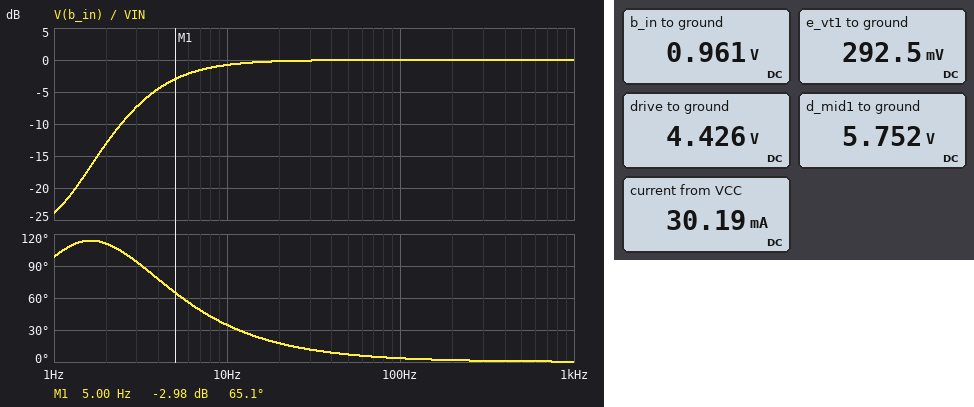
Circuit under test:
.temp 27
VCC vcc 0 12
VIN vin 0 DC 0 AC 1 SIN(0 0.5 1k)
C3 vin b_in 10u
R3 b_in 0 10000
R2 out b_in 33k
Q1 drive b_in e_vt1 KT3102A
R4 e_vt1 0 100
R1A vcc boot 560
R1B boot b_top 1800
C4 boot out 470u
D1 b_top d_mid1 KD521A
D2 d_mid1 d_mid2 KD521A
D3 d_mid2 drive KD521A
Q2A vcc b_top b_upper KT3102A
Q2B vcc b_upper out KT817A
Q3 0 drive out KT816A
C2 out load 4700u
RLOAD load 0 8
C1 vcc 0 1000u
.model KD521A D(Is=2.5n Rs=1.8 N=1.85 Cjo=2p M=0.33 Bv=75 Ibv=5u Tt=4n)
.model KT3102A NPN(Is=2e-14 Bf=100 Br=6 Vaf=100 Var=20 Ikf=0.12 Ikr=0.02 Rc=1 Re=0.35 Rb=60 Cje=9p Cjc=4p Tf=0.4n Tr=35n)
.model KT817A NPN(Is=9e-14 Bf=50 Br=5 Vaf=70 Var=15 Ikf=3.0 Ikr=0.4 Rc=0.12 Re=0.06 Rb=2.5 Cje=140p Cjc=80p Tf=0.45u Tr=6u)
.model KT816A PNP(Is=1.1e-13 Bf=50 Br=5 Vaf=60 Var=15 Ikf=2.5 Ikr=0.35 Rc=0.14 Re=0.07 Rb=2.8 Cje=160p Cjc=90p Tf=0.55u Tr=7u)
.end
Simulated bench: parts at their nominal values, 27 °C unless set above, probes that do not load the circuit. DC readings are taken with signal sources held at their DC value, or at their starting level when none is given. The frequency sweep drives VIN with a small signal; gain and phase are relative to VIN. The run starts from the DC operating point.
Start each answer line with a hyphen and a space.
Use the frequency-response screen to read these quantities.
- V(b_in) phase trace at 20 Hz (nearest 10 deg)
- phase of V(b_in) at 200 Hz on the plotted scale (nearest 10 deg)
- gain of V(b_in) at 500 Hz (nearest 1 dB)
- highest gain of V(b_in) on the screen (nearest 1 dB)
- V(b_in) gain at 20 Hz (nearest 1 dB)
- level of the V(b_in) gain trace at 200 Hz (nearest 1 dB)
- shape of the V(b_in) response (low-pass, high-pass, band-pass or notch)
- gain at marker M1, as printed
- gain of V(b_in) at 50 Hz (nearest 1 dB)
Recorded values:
- 20 deg
- 0 deg
- 0 dB
- 0 dB
- 0 dB
- 0 dB
- high-pass
- -2.98 dB
- 0 dB
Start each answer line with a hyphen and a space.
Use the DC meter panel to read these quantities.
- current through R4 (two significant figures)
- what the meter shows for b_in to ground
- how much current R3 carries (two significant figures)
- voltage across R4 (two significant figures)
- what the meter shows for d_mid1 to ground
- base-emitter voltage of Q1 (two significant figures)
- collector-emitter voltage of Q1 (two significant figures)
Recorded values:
- 2.9 mA
- 0.961 V
- 96 µA
- 290 mV
- 5.752 V
- 670 mV
- 4.1 V
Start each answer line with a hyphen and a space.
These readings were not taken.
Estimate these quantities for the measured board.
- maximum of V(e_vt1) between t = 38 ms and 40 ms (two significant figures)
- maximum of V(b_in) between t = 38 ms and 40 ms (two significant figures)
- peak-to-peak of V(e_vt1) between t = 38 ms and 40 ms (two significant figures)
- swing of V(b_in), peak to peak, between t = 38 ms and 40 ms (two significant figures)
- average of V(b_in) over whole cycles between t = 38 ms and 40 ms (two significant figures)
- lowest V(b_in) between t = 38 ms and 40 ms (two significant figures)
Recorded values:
- 900 mV
- 1.6 V
- 880 mV
- 1.0 V
- 1.1 V
- 600 mV
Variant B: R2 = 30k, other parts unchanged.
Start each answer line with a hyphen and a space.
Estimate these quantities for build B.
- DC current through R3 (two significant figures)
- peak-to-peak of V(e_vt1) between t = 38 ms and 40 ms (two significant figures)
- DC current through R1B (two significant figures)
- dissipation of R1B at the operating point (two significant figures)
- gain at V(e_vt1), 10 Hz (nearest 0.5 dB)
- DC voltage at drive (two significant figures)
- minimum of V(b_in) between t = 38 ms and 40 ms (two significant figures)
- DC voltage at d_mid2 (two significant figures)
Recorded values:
- 98 µA
- 900 mV
- 2.5 mA
- 11 mW
- -1.5 dB
- 4.2 V
- 640 mV
- 4.8 V
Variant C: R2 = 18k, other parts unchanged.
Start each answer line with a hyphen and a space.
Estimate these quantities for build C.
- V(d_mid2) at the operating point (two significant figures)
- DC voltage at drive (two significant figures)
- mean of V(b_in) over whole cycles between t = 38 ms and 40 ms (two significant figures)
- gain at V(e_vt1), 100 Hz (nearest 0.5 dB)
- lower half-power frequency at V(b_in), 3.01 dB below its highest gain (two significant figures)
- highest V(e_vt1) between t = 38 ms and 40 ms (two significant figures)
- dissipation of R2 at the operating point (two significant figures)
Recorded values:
- 3.7 V
- 3.0 V
- 1.3 V
- -0.5 dB
- 7.1 Hz
- 1.1 V
- 380 µW
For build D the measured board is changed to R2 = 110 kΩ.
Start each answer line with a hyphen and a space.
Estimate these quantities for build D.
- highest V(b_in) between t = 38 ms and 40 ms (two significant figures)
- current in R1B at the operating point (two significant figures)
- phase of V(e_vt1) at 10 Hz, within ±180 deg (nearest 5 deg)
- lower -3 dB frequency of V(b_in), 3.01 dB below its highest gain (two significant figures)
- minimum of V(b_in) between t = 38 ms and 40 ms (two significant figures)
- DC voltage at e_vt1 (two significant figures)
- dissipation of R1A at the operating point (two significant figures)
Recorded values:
- 1.2 V
- 680 µA
- 20 deg
- 2.9 Hz
- 180 mV
- 74 mV
- 260 µW
